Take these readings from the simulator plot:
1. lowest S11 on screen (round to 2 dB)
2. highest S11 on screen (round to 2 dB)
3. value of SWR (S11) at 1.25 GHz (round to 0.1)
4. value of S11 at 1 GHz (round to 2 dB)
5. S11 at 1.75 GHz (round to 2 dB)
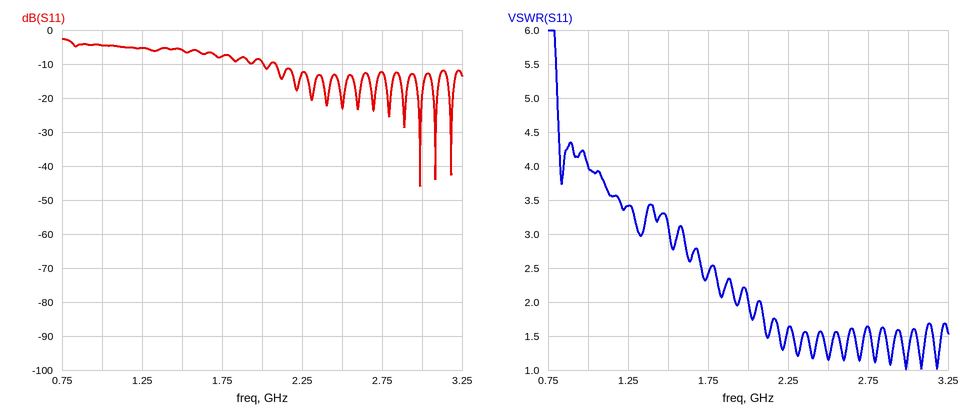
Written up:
-46 dB
-2 dB
3.4
-4 dB
-8 dB
